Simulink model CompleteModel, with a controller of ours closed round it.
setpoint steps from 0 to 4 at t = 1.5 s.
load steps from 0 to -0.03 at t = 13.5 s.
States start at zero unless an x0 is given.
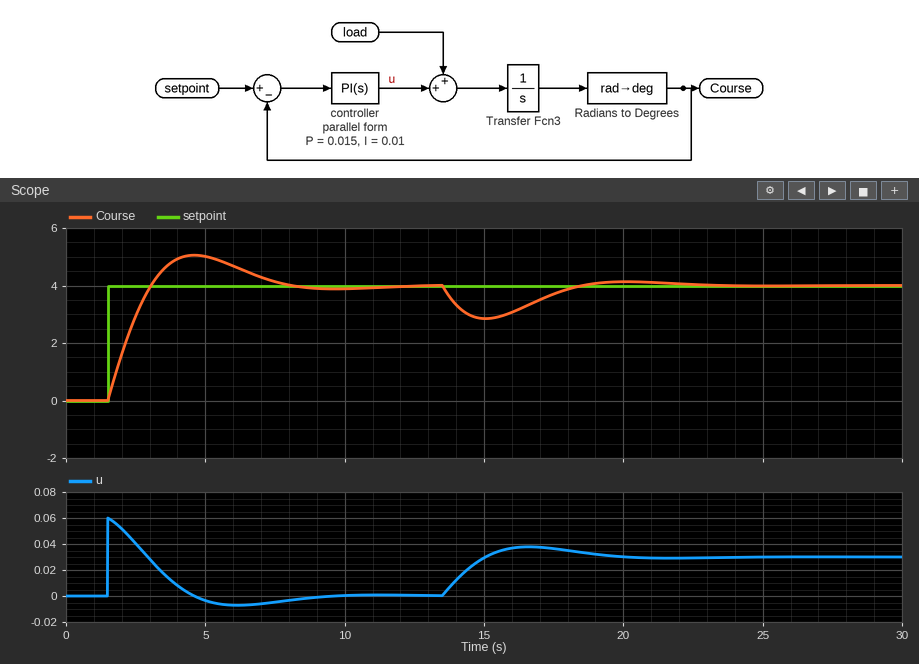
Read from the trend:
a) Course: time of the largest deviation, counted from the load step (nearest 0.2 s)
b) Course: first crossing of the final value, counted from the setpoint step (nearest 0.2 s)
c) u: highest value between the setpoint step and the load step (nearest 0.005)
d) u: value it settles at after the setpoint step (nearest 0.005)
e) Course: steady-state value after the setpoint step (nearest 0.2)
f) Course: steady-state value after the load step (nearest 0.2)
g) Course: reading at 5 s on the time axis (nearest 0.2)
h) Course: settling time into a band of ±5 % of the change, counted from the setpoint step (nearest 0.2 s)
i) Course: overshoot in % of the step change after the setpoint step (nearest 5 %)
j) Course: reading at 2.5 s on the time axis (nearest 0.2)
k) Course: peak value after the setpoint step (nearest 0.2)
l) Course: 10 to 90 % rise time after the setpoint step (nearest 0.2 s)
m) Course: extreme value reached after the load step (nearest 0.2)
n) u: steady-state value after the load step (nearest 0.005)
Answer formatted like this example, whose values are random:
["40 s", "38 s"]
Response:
["1.6 s", "1.6 s", "0.060", "0.000", "4.0", "4.0", "5.0", "5.8 s", "25 %", "3.0", "5.0", "1.2 s", "2.8", "0.030"]
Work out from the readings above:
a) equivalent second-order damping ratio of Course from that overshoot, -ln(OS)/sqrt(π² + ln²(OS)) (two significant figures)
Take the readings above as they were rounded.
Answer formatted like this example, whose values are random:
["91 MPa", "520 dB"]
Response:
["0.40"]
